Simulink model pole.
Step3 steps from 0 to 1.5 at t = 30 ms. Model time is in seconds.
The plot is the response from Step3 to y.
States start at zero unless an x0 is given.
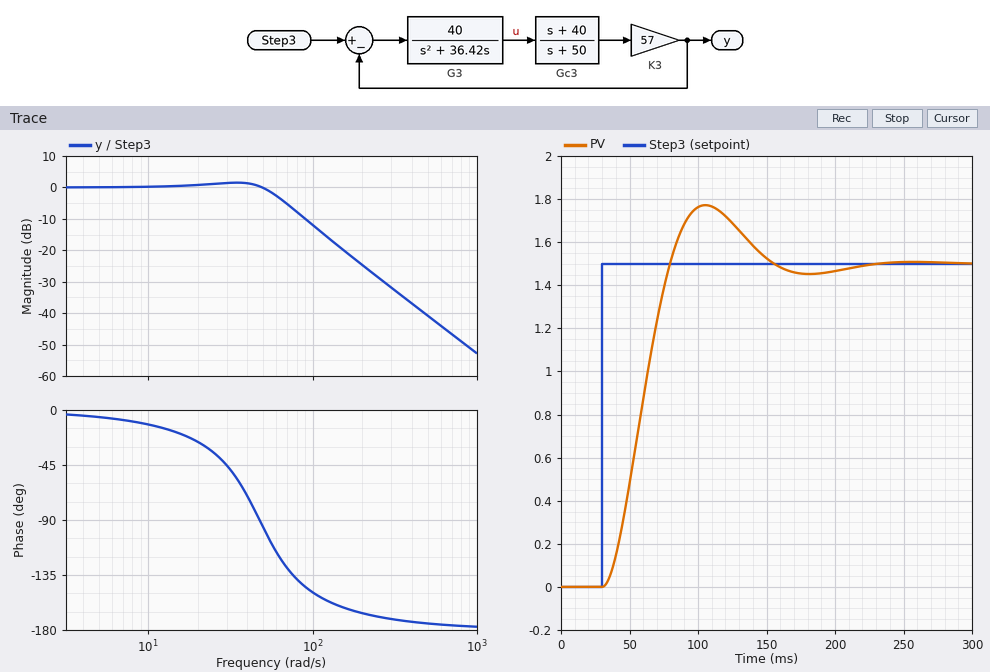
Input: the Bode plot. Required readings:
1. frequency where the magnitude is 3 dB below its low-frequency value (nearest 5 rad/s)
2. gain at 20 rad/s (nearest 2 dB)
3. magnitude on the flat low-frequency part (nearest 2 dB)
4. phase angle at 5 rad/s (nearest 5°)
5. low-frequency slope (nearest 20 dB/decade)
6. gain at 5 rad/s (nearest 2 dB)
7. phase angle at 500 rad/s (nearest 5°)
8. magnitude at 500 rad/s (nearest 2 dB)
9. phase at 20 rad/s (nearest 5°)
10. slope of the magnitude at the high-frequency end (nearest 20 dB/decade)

60 rad/s
0 dB
0 dB
-5°
0 dB/decade
0 dB
-175°
-40 dB
-25°
-40 dB/decade
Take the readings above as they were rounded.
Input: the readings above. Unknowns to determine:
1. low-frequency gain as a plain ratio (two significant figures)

1.0
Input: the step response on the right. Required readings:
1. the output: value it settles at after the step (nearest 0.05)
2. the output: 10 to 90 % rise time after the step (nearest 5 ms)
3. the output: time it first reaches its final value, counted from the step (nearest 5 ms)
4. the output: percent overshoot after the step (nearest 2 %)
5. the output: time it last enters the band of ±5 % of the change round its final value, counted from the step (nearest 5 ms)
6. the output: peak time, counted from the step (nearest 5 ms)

1.50
35 ms
50 ms
18 %
110 ms
75 ms
